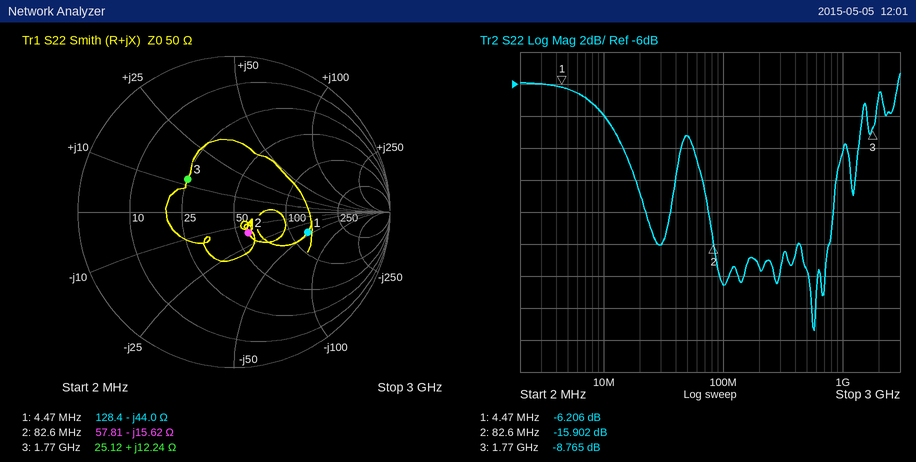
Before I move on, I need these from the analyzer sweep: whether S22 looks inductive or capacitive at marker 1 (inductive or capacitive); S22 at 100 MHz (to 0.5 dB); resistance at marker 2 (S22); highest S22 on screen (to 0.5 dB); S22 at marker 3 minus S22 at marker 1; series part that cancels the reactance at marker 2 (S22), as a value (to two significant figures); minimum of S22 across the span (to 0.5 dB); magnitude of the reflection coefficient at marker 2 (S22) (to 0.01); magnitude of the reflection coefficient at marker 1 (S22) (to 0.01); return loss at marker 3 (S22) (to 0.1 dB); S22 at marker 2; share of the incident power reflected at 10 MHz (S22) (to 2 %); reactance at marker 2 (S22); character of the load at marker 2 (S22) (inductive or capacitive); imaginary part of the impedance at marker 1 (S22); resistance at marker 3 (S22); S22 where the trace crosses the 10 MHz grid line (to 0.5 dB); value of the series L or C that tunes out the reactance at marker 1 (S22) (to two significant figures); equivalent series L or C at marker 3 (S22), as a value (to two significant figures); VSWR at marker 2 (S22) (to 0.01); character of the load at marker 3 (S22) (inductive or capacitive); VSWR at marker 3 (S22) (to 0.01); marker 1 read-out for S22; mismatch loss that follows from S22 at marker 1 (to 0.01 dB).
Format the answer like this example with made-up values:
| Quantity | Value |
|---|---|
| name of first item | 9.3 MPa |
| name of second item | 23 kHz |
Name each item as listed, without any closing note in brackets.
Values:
| Quantity | Value |
|---|---|
| whether S22 looks inductive or capacitive at marker 1 | capacitive |
| S22 at 100 MHz | -18.5 dB |
| resistance at marker 2 | 57.81 Ω |
| highest S22 on screen | -5.5 dB |
| S22 at marker 3 minus S22 at marker 1 | -2.559 dB |
| series part that cancels the reactance at marker 2 (S22), as a value | 30 nH |
| minimum of S22 across the span | -21.5 dB |
| magnitude of the reflection coefficient at marker 2 (S22) | 0.16 |
| magnitude of the reflection coefficient at marker 1 (S22) | 0.49 |
| return loss at marker 3 (S22) | 8.8 dB |
| S22 at marker 2 | -15.902 dB |
| share of the incident power reflected at 10 MHz (S22) | 16 % |
| reactance at marker 2 | -15.62 Ω |
| character of the load at marker 2 (S22) | capacitive |
| imaginary part of the impedance at marker 1 | -44.0 Ω |
| resistance at marker 3 | 25.12 Ω |
| S22 where the trace crosses the 10 MHz grid line | -8.0 dB |
| value of the series L or C that tunes out the reactance at marker 1 (S22) | 1.6 µH |
| equivalent series L or C at marker 3 (S22), as a value | 1.1 nH |
| VSWR at marker 2 (S22) | 1.38 |
| character of the load at marker 3 (S22) | inductive |
| VSWR at marker 3 (S22) | 2.15 |
| marker 1 read-out for S22 | -6.206 dB |
| mismatch loss that follows from S22 at marker 1 | 1.19 dB |
